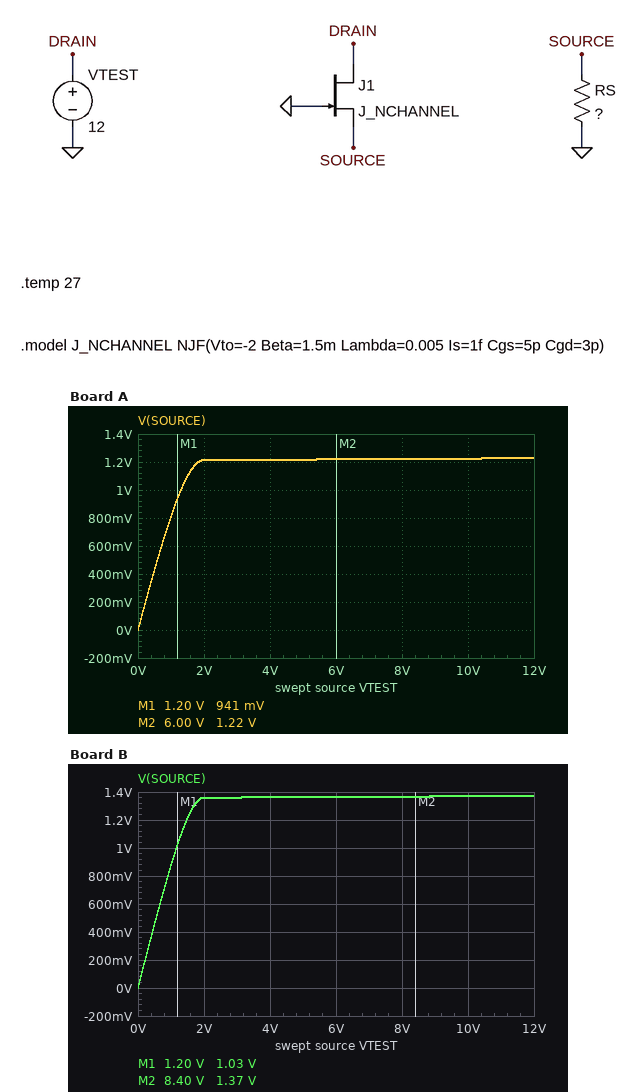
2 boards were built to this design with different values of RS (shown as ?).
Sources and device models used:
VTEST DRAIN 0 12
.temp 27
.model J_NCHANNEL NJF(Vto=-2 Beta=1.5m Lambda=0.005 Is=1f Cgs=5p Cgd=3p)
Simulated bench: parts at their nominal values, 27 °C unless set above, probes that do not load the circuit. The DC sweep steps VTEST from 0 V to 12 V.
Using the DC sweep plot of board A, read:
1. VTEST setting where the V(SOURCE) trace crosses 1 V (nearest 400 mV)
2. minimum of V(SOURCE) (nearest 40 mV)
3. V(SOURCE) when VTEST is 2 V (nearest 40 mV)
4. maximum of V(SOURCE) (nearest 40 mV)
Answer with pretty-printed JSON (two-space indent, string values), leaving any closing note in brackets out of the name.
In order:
{
  "VTEST setting where the V(SOURCE) trace crosses 1 V": "1.2 V",
  "minimum of V(SOURCE)": "0 V",
  "V(SOURCE) when VTEST is 2 V": "1.20 V",
  "maximum of V(SOURCE)": "1.24 V"
}
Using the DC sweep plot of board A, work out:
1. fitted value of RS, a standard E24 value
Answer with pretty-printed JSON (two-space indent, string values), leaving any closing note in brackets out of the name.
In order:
{
  "fitted value of RS, a standard E24 value": "1.3 kΩ"
}
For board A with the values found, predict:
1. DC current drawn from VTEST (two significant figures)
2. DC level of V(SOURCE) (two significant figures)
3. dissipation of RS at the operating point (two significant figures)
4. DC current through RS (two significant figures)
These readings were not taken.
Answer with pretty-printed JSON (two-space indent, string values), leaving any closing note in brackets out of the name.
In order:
{
  "DC current drawn from VTEST": "940 µA",
  "DC level of V(SOURCE)": "1.2 V",
  "dissipation of RS at the operating point": "1.2 mW",
  "DC current through RS": "940 µA"
}
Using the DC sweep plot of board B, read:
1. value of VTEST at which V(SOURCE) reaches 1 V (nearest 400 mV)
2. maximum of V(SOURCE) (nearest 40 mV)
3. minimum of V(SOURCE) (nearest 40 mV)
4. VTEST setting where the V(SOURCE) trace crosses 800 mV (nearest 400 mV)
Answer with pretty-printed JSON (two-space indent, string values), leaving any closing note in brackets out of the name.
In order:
{
  "value of VTEST at which V(SOURCE) reaches 1 V": "1.2 V",
  "maximum of V(SOURCE)": "1.36 V",
  "minimum of V(SOURCE)": "0 V",
  "VTEST setting where the V(SOURCE) trace crosses 800 mV": "800 mV"
}
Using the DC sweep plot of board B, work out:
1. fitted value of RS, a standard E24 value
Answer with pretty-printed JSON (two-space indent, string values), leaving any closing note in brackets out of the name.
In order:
{
  "fitted value of RS, a standard E24 value": "2.2 kΩ"
}
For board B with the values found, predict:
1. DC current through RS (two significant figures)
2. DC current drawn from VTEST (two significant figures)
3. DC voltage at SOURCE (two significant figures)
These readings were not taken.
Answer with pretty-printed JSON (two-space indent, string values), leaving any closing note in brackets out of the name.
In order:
{
  "DC current through RS": "620 µA",
  "DC current drawn from VTEST": "620 µA",
  "DC voltage at SOURCE": "1.4 V"
}
